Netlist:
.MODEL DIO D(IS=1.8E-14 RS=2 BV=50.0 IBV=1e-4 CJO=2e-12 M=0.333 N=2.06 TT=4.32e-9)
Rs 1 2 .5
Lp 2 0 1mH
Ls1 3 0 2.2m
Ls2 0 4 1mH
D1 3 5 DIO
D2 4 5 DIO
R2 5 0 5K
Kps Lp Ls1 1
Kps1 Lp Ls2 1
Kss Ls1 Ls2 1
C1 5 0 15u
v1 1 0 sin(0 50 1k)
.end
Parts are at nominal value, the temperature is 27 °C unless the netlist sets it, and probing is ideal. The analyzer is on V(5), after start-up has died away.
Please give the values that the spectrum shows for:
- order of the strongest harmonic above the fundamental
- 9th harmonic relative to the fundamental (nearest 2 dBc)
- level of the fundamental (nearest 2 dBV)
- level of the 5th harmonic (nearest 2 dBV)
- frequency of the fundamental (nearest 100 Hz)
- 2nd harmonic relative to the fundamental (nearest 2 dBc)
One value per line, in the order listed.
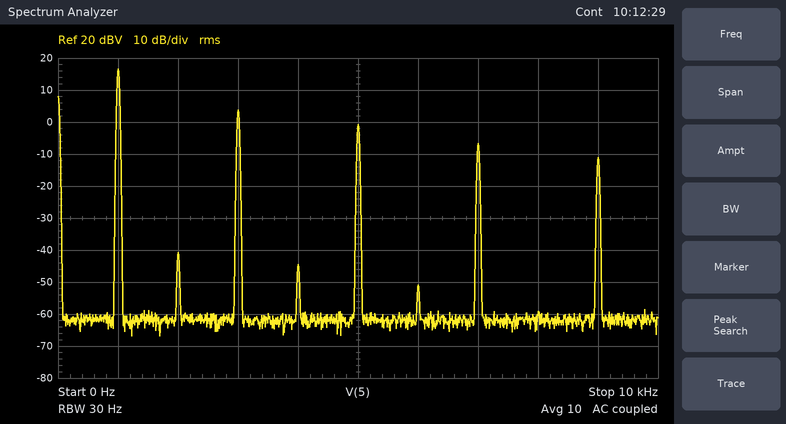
3
-28 dBc
16 dBV
0 dBV
1.0 kHz
-58 dBc
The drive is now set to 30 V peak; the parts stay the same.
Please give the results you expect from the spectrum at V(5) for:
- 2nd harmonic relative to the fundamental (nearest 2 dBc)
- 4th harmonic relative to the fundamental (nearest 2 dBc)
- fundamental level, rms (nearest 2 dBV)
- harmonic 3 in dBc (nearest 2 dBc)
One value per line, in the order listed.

-48 dBc
-58 dBc
14 dBV
-10 dBc
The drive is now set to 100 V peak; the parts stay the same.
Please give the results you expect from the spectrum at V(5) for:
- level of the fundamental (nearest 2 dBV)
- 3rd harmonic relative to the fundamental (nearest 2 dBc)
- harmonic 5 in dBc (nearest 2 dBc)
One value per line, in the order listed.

22 dBV
-20 dBc
-22 dBc
